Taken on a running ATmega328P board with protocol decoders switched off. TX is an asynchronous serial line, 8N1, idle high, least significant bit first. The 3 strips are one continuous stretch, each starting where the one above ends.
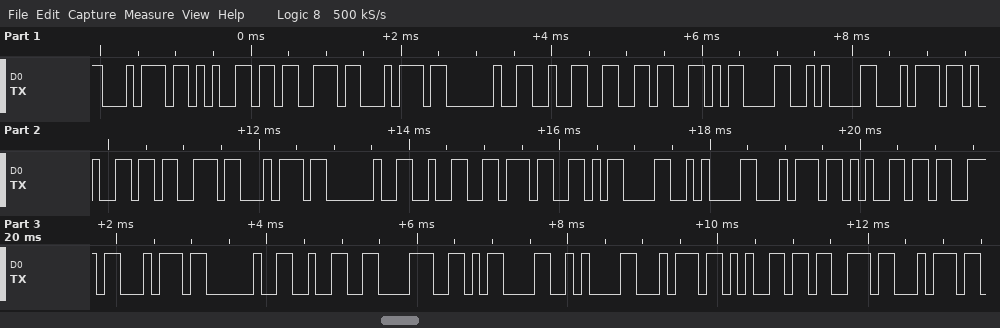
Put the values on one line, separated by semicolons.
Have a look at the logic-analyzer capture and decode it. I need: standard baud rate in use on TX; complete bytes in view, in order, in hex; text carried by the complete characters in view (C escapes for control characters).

9600 baud; 74 65 73 74 20 32 36 0D 0A 74 65 73 74 20 32 37 0D 0A 74 65 73 74 20 32 38 0D 0A 74 65 73 74; "test 26\r\ntest 27\r\ntest 28\r\ntest"
